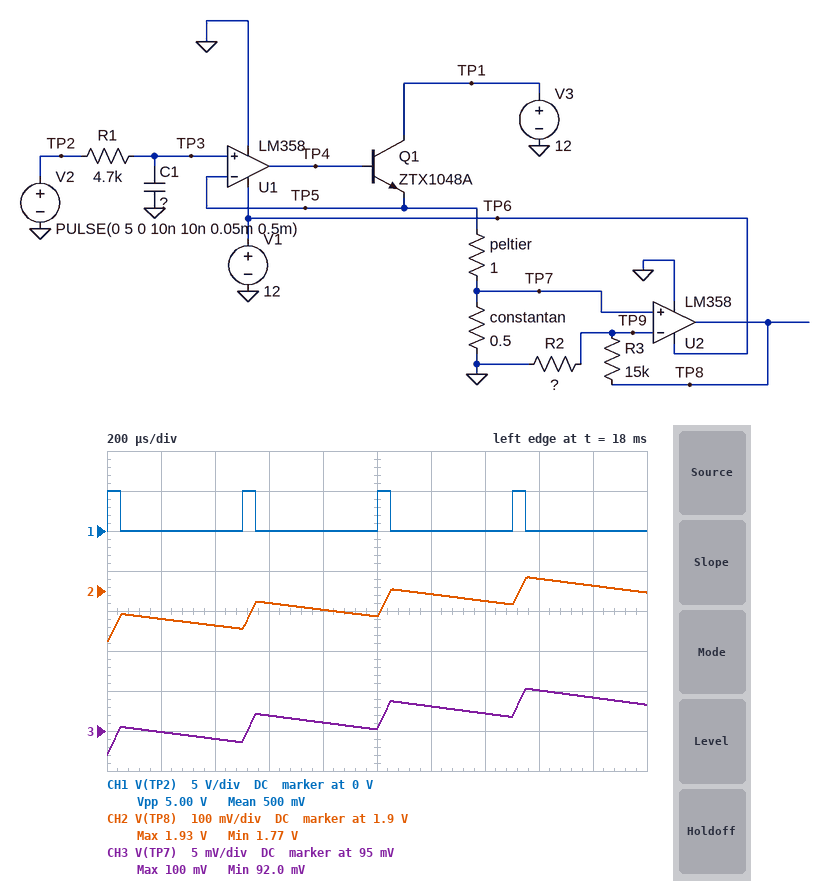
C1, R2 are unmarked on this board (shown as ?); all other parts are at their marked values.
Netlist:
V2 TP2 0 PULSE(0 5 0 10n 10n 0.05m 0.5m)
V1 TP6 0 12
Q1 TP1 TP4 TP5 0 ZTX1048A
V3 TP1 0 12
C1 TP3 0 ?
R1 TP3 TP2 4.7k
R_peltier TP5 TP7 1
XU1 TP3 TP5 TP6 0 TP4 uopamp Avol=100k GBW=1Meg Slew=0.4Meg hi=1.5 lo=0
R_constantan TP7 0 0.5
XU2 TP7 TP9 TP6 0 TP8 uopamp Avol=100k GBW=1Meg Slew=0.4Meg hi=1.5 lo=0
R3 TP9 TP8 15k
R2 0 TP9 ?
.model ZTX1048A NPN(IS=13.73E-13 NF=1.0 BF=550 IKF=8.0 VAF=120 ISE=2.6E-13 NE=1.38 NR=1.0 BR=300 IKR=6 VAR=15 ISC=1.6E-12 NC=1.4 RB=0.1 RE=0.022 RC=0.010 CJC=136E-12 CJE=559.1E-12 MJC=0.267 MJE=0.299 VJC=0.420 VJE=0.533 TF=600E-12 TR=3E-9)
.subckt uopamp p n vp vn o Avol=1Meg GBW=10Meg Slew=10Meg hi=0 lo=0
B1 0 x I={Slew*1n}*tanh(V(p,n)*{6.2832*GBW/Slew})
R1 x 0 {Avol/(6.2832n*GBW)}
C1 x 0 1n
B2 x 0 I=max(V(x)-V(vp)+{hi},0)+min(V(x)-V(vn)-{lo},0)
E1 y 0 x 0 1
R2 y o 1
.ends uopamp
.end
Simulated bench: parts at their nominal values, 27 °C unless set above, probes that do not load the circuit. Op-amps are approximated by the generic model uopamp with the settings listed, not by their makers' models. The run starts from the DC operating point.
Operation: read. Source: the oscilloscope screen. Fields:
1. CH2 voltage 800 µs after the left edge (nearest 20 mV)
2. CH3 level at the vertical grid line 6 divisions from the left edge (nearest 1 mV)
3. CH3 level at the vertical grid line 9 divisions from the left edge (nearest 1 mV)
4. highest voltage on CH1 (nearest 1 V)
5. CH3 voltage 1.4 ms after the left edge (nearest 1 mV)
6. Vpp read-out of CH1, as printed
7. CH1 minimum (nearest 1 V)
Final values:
1.86 V
98 mV
99 mV
5 V
97 mV
5.00 V
0 V
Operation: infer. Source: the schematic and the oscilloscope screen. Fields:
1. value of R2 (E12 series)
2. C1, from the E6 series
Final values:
820 Ω
4.7 µF
